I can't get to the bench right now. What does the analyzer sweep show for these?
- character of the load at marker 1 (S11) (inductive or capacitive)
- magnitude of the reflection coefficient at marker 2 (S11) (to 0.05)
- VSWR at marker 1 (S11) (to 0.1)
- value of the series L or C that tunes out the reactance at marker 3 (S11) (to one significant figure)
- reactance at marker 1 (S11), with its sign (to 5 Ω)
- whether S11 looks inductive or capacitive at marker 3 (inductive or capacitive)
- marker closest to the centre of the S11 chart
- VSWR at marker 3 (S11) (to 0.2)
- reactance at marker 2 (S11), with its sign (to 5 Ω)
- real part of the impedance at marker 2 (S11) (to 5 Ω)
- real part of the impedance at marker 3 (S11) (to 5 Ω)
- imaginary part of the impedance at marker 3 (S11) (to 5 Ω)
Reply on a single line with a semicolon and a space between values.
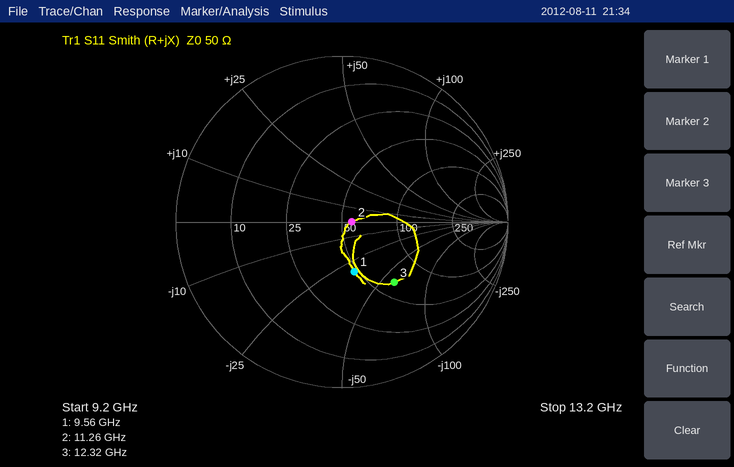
capacitive; 0.05; 1.9; 800 pH; -30 Ω; capacitive; marker 2; 2.8; 0 Ω; 55 Ω; 65 Ω; -60 Ω
